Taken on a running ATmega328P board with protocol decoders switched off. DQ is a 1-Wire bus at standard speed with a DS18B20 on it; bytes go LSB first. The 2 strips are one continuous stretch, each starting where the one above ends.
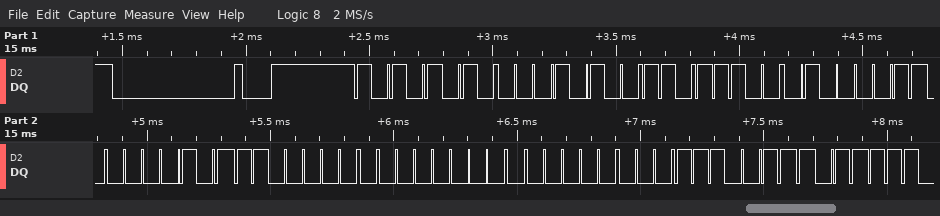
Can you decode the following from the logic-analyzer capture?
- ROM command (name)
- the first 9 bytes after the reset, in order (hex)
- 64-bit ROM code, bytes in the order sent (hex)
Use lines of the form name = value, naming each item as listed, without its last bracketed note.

ROM command = Match ROM
the first 9 bytes after the reset, in order = 55 28 3B C2 A0 03 00 00 E7
64-bit ROM code, bytes in the order sent = 28 3B C2 A0 03 00 00 E7
